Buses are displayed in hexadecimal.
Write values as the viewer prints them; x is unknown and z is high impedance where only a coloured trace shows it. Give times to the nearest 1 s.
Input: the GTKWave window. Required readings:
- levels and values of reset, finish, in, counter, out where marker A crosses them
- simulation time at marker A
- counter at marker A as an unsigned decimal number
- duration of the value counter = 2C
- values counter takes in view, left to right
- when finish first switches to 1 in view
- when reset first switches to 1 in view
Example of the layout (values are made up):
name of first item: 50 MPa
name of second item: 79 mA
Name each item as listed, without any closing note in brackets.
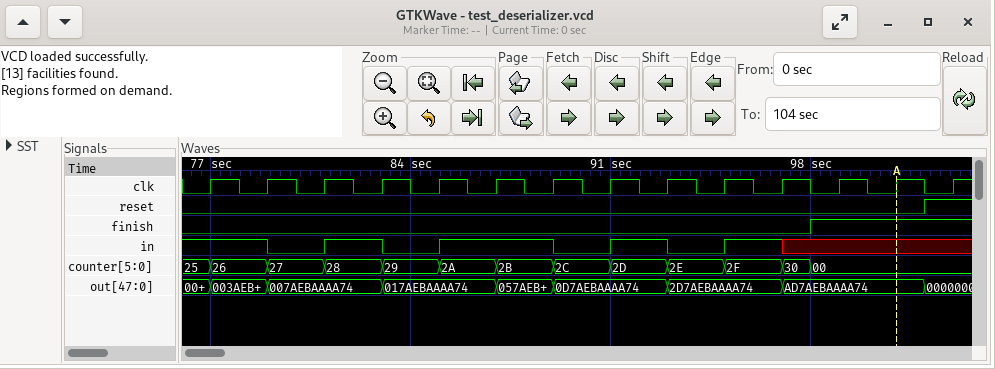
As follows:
levels and values of reset, finish, in, counter, out where marker A crosses them: reset=0, finish=1, in=x, counter=00, out=AD7AEBAAAA74
simulation time at marker A: 101 s
counter at marker A as an unsigned decimal number: 0
duration of the value counter = 2C: 2 s
values counter takes in view, left to right: 25, 26, 27, 28, 29, 2A, 2B, 2C, 2D, 2E, 2F, 30, 00
when finish first switches to 1 in view: 98 s
when reset first switches to 1 in view: 102 s
